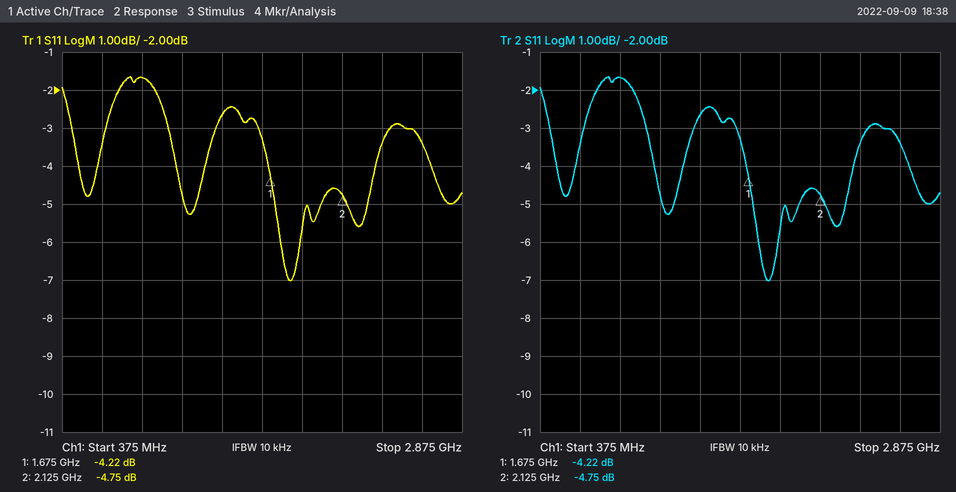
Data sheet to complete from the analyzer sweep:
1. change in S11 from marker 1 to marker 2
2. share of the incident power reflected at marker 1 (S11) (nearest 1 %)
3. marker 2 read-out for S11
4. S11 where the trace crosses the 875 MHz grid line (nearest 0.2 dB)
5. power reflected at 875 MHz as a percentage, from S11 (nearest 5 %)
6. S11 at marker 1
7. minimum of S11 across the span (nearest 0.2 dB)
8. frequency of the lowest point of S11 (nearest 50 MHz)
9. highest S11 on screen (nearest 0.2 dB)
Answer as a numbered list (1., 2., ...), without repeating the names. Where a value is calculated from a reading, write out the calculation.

1. -4.75 − (-4.22) = -0.53 dB
2. 10^(-4.22/10) ≈ 38 %
3. -4.75 dB
4. -1.6 dB
5. 10^(-1.6/10) ≈ 69.2 %, so 70 % to the nearest 5 %
6. -4.22 dB
7. -7.0 dB
8. 1.80 GHz
9. -1.6 dB
